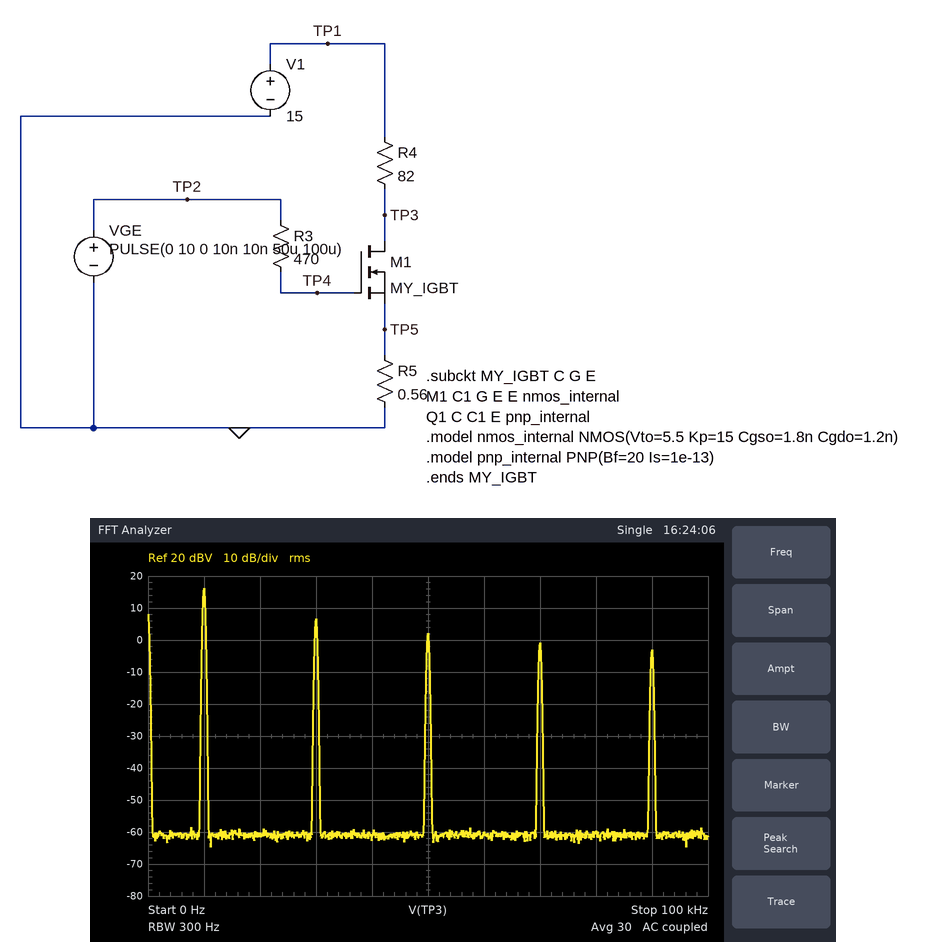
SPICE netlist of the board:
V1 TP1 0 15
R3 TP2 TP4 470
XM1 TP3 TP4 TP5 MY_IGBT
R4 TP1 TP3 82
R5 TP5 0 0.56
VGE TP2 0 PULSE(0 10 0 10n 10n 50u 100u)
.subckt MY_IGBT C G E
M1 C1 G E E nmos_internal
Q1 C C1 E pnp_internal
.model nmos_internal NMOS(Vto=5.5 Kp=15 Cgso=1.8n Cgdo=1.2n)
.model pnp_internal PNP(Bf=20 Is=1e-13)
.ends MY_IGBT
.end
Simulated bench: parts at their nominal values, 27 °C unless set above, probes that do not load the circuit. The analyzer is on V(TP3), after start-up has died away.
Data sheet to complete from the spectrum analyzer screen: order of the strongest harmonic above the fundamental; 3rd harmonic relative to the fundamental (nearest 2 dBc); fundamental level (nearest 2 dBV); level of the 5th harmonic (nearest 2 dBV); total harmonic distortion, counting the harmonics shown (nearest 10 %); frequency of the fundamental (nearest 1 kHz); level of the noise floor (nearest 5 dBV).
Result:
3
-10 dBc
16 dBV
2 dBV
40 %
10 kHz
-60 dBV
